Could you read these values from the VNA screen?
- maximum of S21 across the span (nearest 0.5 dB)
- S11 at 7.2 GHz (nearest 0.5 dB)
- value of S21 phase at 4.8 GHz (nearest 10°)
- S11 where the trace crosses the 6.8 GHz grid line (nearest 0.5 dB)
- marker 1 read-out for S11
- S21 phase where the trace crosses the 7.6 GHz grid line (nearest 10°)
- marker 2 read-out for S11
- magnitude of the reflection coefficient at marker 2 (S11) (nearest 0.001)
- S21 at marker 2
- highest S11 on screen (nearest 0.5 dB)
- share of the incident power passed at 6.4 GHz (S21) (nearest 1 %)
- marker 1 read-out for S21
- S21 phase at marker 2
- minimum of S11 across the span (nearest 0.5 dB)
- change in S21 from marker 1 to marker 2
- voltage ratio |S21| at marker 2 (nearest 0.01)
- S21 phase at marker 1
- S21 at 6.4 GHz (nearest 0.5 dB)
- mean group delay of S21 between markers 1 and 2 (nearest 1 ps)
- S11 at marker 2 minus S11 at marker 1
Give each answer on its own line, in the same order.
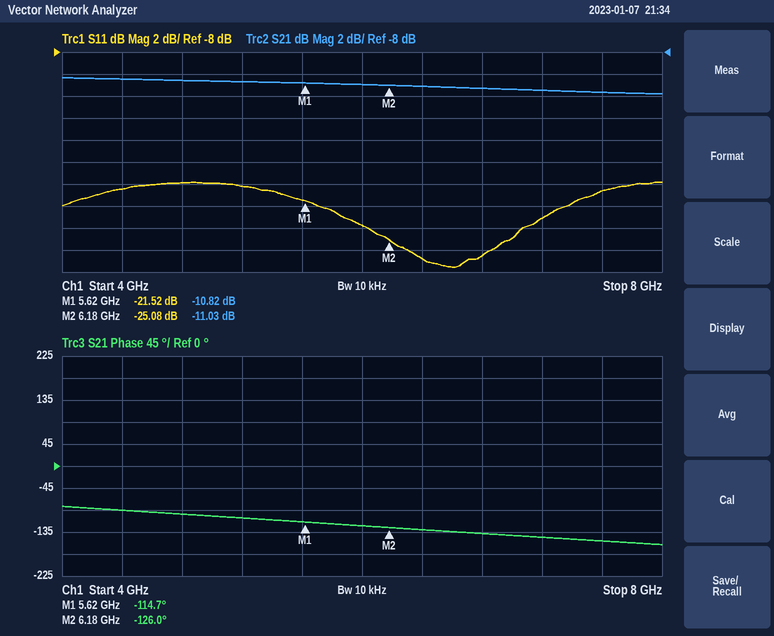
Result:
-10.5 dB
-23.0 dB
-100°
-26.5 dB
-21.52 dB
-150°
-25.08 dB
0.056
-11.03 dB
-20.0 dB
8 %
-10.82 dB
-126.0°
-27.5 dB
-0.21 dB
0.28
-114.7°
-11.0 dB
56 ps
-3.56 dB
